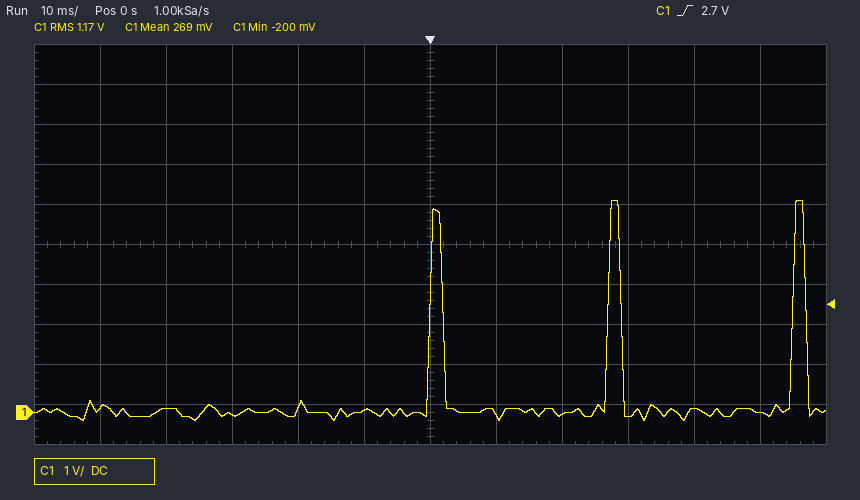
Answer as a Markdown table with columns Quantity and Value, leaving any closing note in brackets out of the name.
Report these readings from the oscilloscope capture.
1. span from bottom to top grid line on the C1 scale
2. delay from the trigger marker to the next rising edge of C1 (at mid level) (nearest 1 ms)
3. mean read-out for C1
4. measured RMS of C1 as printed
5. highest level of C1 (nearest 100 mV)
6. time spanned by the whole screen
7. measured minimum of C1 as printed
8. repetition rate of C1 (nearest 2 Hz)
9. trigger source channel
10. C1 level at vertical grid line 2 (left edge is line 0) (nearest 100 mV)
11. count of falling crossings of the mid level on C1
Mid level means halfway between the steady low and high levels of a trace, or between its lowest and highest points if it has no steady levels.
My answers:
| Quantity | Value |
|---|---|
| span from bottom to top grid line on the C1 scale | 10 V |
| delay from the trigger marker to the next rising edge of C1 (at mid level) | 27 ms |
| mean read-out for C1 | 269 mV |
| measured RMS of C1 as printed | 1.17 V |
| highest level of C1 | 5.3 V |
| time spanned by the whole screen | 120 ms |
| measured minimum of C1 as printed | -200 mV |
| repetition rate of C1 | 36 Hz |
| trigger source channel | C1 |
| C1 level at vertical grid line 2 (left edge is line 0) | 100 mV |
| count of falling crossings of the mid level on C1 | 3 |
